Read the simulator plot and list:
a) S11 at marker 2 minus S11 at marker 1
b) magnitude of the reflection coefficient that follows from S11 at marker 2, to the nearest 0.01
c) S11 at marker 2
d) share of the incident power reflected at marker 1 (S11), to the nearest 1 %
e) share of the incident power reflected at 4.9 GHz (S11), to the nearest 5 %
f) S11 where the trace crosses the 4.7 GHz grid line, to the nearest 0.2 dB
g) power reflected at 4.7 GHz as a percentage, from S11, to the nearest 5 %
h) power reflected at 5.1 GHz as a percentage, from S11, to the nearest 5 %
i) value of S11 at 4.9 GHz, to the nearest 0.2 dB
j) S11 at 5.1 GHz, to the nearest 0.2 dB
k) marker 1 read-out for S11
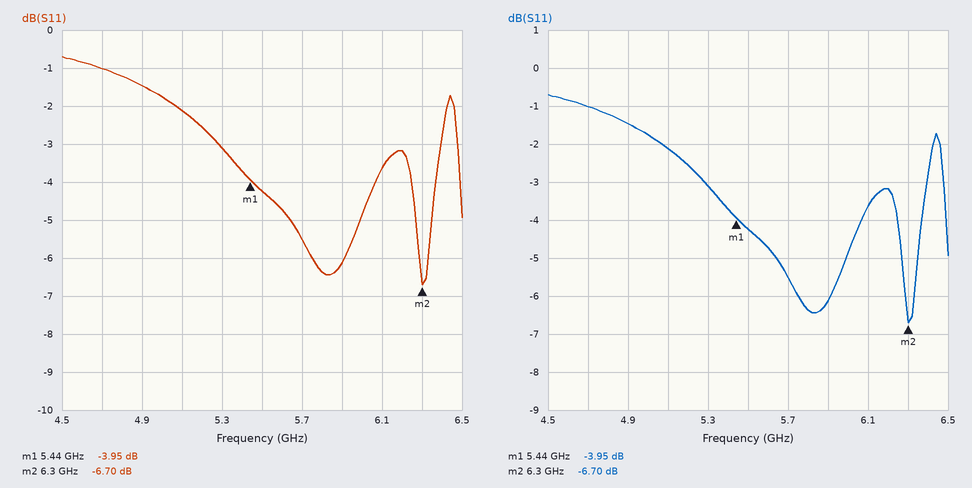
-2.75 dB
0.46
-6.70 dB
40 %
70 %
-1.0 dB
80 %
60 %
-1.4 dB
-2.2 dB
-3.95 dB
